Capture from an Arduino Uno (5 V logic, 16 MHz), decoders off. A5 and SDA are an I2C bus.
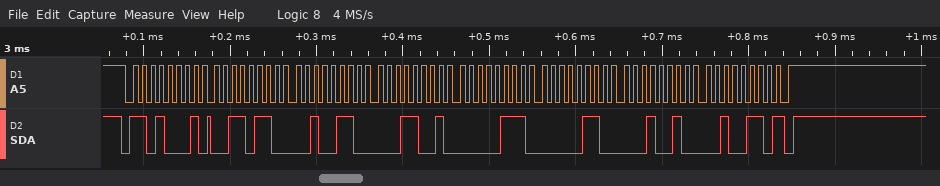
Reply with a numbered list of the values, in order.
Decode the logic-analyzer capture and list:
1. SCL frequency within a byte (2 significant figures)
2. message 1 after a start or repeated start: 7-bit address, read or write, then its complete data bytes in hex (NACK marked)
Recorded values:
1. 100 kHz
2. 0x68 read: 36 26 19 07 06 12 26 NACK
